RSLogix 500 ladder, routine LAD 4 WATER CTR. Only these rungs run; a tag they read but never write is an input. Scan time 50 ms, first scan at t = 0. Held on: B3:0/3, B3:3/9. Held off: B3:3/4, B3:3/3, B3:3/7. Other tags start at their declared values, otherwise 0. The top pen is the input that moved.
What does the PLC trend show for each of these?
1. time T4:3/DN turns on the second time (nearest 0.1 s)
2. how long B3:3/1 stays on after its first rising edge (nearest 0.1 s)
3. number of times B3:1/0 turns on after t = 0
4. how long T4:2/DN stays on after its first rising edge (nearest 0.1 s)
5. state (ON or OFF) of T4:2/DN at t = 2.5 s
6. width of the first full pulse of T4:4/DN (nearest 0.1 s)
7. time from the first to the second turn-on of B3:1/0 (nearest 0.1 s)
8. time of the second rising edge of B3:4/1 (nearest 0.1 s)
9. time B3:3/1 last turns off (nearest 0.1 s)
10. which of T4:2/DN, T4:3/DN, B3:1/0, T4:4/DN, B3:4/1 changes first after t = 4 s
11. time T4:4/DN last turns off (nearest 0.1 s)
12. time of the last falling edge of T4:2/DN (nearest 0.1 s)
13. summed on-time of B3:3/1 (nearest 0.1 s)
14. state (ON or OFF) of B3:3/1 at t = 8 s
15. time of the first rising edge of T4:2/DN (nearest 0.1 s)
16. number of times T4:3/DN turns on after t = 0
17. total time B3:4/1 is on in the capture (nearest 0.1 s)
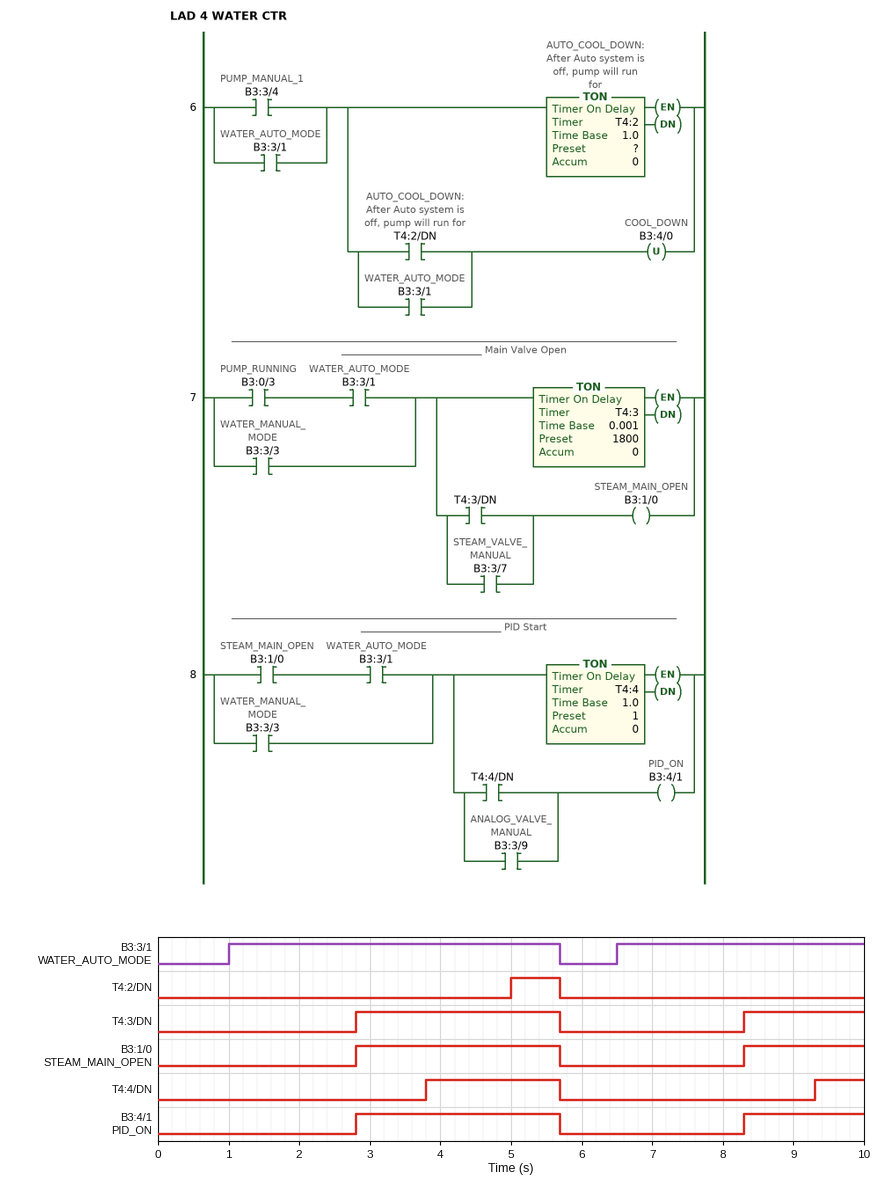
8.3 s
4.7 s
2
0.7 s
OFF
1.9 s
5.5 s
8.3 s
5.7 s
T4:2/DN
5.7 s
5.7 s
8.2 s
ON
5.0 s
2
4.6 s
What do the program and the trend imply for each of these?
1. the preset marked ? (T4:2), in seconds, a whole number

4 s
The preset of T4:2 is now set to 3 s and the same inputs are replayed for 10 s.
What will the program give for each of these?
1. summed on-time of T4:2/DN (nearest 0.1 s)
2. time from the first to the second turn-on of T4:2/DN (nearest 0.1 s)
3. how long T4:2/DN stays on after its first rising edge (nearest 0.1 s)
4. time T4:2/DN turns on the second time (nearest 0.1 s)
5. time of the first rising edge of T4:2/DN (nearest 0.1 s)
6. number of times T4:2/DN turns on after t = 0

2.2 s
5.5 s
1.7 s
9.5 s
4.0 s
2
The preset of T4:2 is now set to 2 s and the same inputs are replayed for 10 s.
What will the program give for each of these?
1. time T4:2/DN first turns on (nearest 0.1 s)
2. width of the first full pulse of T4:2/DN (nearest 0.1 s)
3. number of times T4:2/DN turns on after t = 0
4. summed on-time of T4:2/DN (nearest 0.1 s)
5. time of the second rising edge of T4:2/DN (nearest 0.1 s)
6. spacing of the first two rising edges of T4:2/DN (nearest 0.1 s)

3.0 s
2.7 s
2
4.2 s
8.5 s
5.5 s
